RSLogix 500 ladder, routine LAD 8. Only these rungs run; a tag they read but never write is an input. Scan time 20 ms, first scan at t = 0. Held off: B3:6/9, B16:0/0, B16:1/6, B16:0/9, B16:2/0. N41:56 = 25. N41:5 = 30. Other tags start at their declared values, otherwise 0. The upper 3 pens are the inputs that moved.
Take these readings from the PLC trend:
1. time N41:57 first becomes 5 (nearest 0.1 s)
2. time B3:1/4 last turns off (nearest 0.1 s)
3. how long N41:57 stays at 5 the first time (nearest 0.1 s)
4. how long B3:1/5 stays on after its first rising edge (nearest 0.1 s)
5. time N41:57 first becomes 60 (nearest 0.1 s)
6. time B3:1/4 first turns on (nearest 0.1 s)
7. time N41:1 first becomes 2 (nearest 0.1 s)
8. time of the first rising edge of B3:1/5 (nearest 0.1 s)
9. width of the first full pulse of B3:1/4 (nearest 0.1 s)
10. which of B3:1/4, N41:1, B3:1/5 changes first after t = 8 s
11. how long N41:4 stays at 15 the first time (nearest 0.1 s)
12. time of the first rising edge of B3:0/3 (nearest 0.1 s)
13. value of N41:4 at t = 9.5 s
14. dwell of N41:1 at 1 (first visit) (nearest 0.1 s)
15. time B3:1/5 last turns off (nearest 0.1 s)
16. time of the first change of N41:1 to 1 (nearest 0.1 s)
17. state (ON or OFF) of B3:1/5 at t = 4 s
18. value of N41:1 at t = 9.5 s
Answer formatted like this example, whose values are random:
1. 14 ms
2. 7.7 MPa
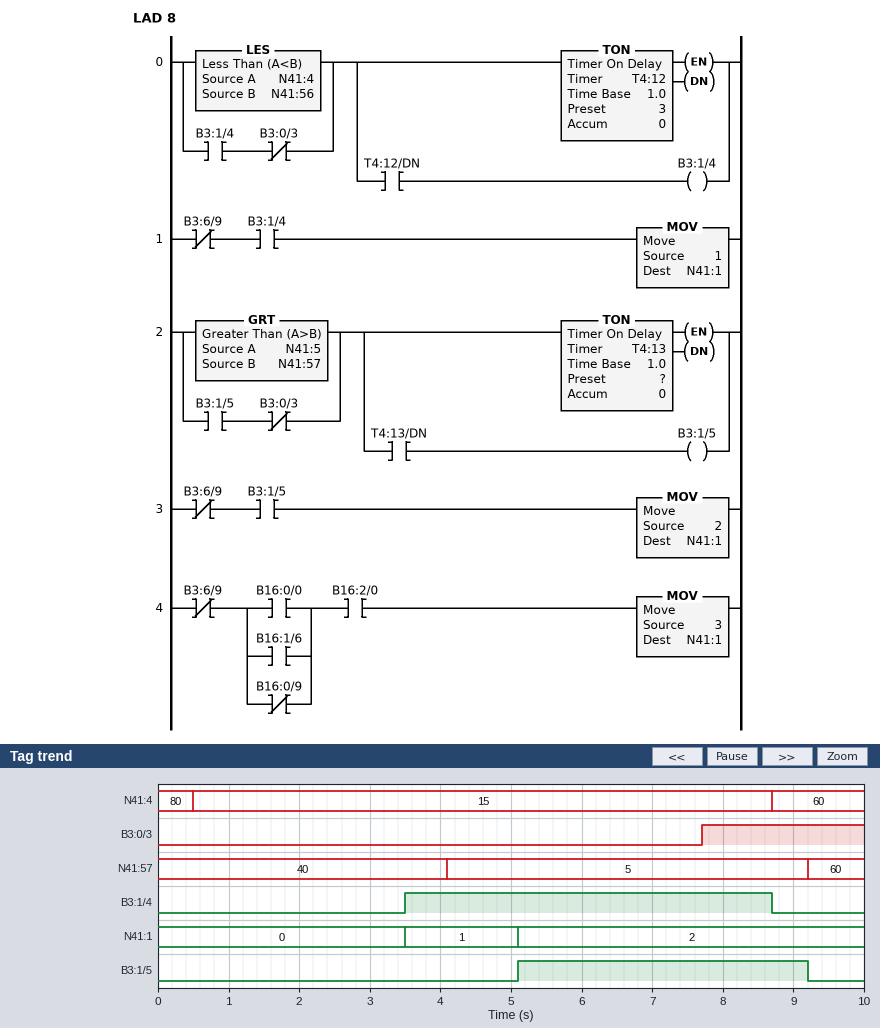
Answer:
1. 4.1 s
2. 8.7 s
3. 5.1 s
4. 4.1 s
5. 9.2 s
6. 3.5 s
7. 5.1 s
8. 5.1 s
9. 5.2 s
10. B3:1/4
11. 8.2 s
12. 7.7 s
13. 60
14. 1.6 s
15. 9.2 s
16. 3.5 s
17. OFF
18. 2
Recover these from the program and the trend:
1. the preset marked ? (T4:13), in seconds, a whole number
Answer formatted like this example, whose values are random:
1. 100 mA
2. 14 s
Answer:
1. 1 s
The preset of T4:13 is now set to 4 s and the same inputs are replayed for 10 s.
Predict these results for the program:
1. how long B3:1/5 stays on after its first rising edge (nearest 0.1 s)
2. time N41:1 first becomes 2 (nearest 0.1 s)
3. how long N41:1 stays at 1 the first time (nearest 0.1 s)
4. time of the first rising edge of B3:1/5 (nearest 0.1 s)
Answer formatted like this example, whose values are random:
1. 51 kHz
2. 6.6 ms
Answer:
1. 1.1 s
2. 8.1 s
3. 4.6 s
4. 8.1 s
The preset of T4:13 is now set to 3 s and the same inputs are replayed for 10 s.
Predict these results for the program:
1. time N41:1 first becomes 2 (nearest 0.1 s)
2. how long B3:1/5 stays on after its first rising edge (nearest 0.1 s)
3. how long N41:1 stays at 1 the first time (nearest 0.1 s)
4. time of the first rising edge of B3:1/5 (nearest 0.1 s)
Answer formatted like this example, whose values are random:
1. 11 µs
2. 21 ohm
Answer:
1. 7.1 s
2. 2.1 s
3. 3.6 s
4. 7.1 s
